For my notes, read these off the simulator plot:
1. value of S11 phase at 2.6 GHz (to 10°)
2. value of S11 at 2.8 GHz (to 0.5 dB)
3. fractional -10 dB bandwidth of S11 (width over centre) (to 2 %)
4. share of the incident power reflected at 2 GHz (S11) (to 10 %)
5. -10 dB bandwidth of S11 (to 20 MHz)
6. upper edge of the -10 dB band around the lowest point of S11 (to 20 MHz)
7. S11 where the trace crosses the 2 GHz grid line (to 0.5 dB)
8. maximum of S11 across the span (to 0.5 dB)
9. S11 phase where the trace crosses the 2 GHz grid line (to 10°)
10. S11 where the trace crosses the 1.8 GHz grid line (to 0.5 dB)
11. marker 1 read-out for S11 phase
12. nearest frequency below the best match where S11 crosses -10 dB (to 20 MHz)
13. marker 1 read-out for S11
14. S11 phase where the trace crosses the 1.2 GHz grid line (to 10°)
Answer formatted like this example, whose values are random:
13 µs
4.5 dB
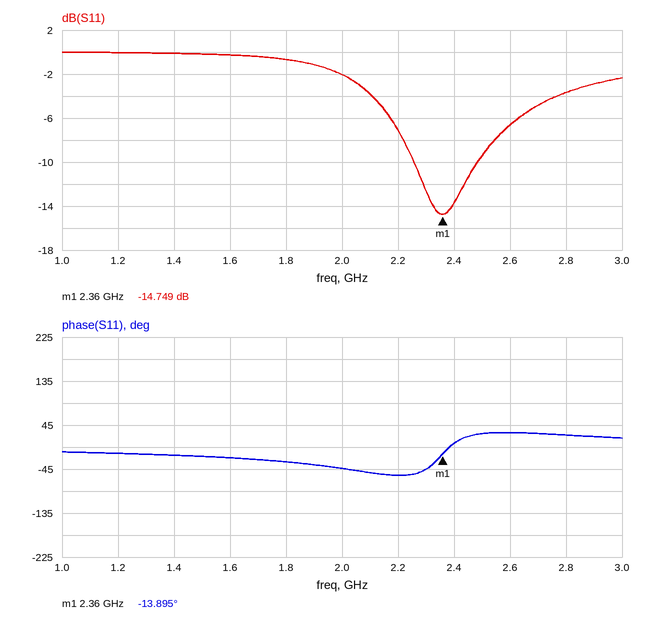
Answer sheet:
30°
-3.5 dB
10 %
60 %
220 MHz
2.48 GHz
-2.0 dB
0.0 dB
-40°
-0.5 dB
-13.895°
2.26 GHz
-14.749 dB
-10°
